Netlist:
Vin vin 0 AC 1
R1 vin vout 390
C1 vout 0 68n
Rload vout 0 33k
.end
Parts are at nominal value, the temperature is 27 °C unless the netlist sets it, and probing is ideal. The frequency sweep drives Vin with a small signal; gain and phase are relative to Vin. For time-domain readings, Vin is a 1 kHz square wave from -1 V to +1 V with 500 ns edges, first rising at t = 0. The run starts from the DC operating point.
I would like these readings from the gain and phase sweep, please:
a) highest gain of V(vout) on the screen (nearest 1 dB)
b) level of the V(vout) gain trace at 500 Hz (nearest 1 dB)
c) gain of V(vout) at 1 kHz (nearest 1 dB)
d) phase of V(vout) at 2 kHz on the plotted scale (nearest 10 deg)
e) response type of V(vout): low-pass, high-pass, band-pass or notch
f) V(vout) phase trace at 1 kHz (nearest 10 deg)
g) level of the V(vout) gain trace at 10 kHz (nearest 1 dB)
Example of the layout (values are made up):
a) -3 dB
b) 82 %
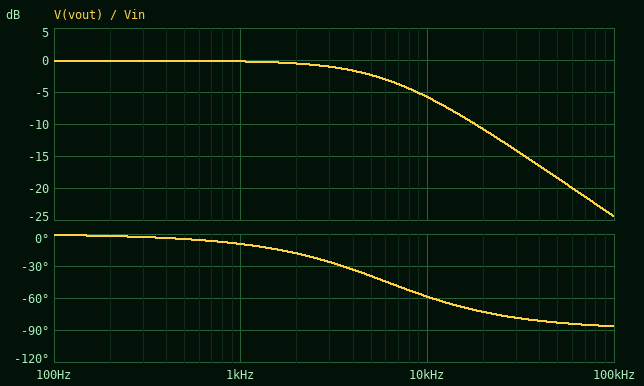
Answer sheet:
a) 0 dB
b) 0 dB
c) 0 dB
d) -20 deg
e) low-pass
f) -10 deg
g) -6 dB
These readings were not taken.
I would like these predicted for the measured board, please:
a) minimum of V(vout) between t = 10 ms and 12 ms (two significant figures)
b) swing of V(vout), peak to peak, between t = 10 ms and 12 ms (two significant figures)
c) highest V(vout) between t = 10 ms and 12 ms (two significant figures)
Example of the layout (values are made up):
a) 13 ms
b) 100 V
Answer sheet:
a) -990 mV
b) 2.0 V
c) 990 mV
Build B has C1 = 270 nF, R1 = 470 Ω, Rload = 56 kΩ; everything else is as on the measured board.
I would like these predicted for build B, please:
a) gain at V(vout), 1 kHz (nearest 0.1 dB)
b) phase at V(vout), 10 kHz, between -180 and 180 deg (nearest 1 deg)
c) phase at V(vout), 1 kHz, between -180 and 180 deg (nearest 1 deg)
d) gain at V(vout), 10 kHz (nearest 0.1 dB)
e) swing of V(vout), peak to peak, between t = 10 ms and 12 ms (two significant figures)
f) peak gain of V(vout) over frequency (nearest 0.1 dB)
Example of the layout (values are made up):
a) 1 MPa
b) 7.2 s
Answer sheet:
a) -2.2 dB
b) -83 deg
c) -38 deg
d) -18.1 dB
e) 1.9 V
f) -0.1 dB
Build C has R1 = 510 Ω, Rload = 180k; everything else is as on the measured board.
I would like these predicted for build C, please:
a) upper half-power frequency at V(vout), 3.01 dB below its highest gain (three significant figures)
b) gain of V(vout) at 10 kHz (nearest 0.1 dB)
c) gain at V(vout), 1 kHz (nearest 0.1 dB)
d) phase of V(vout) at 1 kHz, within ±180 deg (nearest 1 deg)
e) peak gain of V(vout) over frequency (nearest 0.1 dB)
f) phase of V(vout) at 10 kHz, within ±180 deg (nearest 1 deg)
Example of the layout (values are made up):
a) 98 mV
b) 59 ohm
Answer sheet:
a) 4.60 kHz
b) -7.6 dB
c) -0.2 dB
d) -12 deg
e) 0 dB
f) -65 deg
